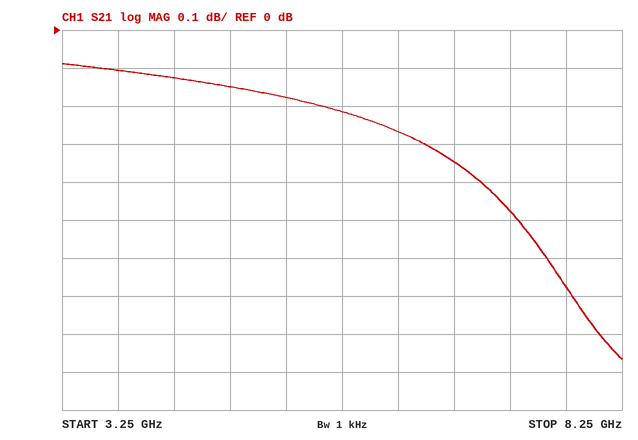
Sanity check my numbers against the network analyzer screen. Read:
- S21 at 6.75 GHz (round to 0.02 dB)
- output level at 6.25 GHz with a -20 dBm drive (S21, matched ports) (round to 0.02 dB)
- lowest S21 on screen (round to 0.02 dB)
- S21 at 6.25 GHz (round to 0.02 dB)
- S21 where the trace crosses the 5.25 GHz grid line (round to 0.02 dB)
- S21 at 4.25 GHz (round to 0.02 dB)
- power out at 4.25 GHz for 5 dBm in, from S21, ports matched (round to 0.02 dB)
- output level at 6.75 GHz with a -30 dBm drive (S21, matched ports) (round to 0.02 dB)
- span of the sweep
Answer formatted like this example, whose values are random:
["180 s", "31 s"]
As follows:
["-0.34 dB", "-20.26 dBm", "-0.86 dB", "-0.26 dB", "-0.18 dB", "-0.12 dB", "4.88 dBm", "-30.34 dBm", "5 GHz"]
